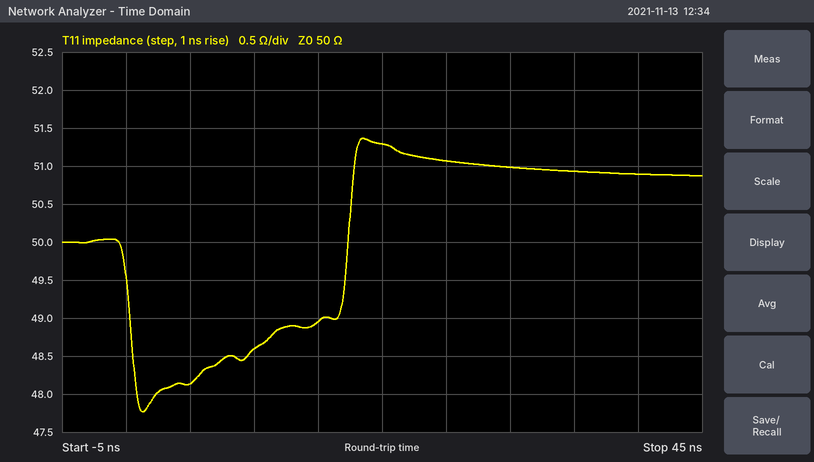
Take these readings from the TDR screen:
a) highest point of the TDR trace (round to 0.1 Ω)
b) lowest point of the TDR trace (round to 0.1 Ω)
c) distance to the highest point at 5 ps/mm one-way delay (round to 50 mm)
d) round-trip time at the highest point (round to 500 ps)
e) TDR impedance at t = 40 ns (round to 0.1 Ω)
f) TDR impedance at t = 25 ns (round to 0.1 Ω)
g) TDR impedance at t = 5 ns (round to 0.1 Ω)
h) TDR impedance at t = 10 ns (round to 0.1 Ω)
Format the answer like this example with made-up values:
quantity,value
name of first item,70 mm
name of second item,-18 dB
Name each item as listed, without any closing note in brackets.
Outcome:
quantity,value
highest point of the TDR trace,51.4 Ω
lowest point of the TDR trace,47.8 Ω
distance to the highest point at 5 ps/mm one-way delay,1.85 m
round-trip time at the highest point,18.5 ns
TDR impedance at t = 40 ns,50.9 Ω
TDR impedance at t = 25 ns,51.1 Ω
TDR impedance at t = 5 ns,48.1 Ω
TDR impedance at t = 10 ns,48.6 Ω
